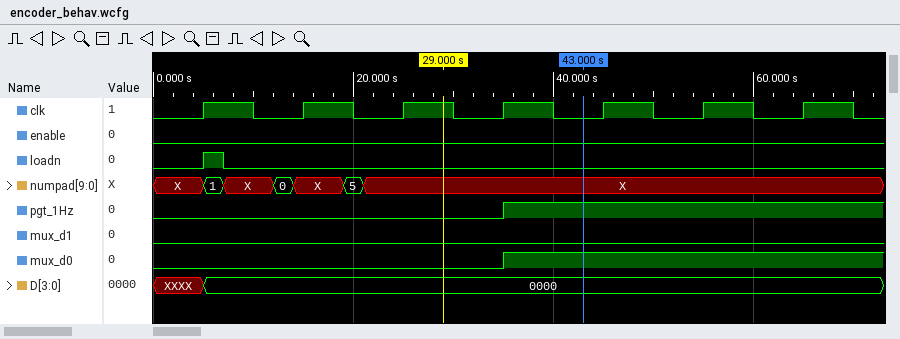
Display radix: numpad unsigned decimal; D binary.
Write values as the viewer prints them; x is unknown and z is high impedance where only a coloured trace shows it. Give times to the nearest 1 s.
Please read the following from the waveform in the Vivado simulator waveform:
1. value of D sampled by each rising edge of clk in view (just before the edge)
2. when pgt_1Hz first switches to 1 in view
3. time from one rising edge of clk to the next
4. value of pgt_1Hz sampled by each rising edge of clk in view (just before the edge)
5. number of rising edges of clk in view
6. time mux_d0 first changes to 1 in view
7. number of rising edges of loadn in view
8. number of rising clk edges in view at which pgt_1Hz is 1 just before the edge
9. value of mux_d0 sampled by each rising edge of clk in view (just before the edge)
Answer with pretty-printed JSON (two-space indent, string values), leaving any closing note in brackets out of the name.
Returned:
{
  "value of D sampled by each rising edge of clk in view": "XXXX, 0000, 0000, 0000, 0000, 0000, 0000",
  "when pgt_1Hz first switches to 1 in view": "35 s",
  "time from one rising edge of clk to the next": "10 s",
  "value of pgt_1Hz sampled by each rising edge of clk in view": "0 0 0 0 1 1 1",
  "number of rising edges of clk in view": "7",
  "time mux_d0 first changes to 1 in view": "35 s",
  "number of rising edges of loadn in view": "1",
  "number of rising clk edges in view at which pgt_1Hz is 1 just before the edge": "3",
  "value of mux_d0 sampled by each rising edge of clk in view": "0 0 0 0 1 1 1"
}
